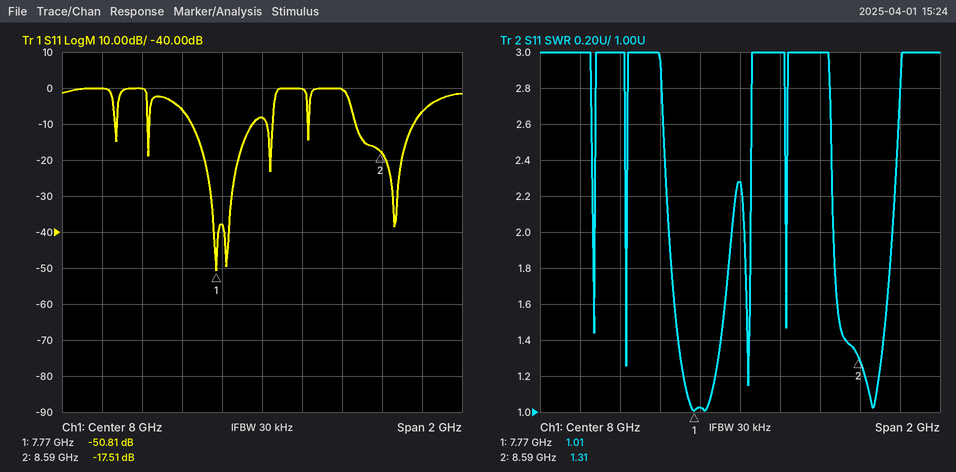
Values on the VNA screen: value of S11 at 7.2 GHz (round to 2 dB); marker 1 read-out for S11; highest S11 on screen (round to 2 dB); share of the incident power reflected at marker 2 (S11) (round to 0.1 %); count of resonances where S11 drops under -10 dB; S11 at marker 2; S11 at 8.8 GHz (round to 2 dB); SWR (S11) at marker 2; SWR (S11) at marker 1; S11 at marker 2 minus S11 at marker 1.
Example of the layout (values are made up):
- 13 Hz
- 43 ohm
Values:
- 0 dB
- -50.81 dB
- 0 dB
- 1.8 %
- 7
- -17.51 dB
- -6 dB
- 1.31
- 1.01
- 33.30 dB
